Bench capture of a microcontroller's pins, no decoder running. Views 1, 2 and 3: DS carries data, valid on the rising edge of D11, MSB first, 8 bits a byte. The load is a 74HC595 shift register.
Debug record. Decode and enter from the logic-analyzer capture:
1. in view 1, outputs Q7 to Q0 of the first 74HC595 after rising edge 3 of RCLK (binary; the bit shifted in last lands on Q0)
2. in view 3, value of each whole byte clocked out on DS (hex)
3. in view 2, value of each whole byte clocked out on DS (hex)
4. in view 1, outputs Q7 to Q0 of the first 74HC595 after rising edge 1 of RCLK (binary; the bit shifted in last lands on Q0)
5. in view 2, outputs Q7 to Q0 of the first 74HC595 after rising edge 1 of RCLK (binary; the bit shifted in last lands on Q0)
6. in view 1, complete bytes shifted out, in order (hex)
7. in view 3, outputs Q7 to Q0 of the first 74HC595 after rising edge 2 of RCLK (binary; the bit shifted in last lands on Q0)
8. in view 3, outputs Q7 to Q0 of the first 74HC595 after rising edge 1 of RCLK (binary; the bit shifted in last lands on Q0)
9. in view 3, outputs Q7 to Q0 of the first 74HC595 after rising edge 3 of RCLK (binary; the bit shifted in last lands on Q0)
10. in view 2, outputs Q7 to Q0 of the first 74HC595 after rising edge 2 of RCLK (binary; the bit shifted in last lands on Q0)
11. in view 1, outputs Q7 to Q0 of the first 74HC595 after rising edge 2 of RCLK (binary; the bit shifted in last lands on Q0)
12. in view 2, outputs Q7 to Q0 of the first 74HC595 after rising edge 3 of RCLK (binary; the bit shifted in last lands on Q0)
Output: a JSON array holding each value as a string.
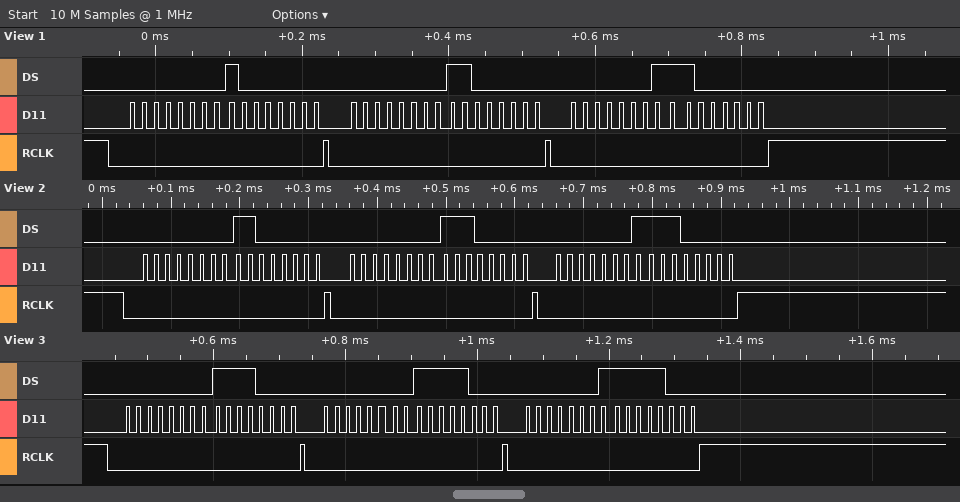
["11000000", "00 F0 00 F8 01 F8", "0x00 0xC0 0x00 0xE0 0x01 0xE0", "10000000", "11000000", "0x00 0x80 0x00 0xC0 0x01 0xC0", "11111000", "11110000", "11111000", "11100000", "11000000", "11100000"]
